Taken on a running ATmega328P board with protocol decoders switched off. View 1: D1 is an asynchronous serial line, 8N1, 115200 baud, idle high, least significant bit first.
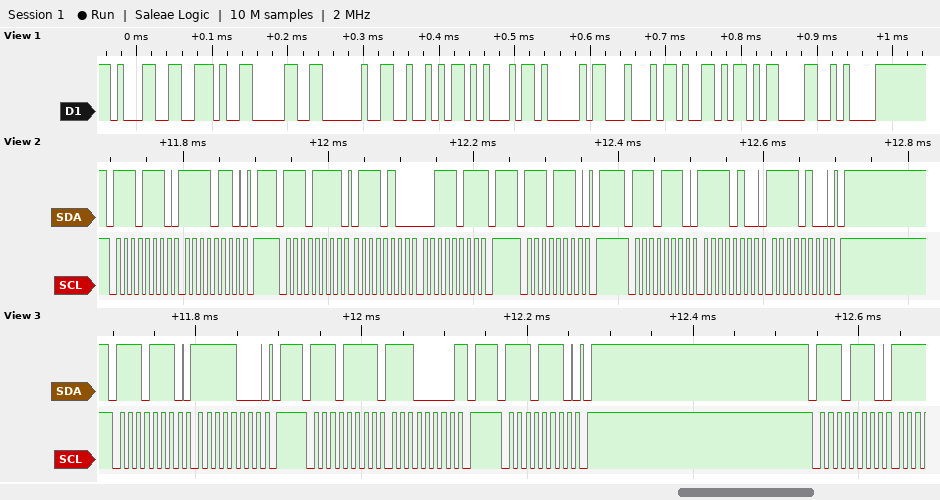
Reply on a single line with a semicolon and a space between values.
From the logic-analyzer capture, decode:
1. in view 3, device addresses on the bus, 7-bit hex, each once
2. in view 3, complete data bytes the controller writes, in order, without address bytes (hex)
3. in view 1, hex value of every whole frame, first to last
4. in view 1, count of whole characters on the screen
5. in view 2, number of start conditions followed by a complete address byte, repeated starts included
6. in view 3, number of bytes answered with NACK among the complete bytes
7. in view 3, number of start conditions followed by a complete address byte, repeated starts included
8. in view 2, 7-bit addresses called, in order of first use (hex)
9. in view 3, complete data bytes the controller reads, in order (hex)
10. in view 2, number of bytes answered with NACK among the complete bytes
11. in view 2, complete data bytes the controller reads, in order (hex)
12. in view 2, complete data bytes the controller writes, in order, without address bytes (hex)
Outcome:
0x77; F8; 31 2E 30 20 52 45 41 44 59 0D 0A; 11; 4; 1; 4; 0x77; E0; 1; 74 3B; F6 F4 F4
